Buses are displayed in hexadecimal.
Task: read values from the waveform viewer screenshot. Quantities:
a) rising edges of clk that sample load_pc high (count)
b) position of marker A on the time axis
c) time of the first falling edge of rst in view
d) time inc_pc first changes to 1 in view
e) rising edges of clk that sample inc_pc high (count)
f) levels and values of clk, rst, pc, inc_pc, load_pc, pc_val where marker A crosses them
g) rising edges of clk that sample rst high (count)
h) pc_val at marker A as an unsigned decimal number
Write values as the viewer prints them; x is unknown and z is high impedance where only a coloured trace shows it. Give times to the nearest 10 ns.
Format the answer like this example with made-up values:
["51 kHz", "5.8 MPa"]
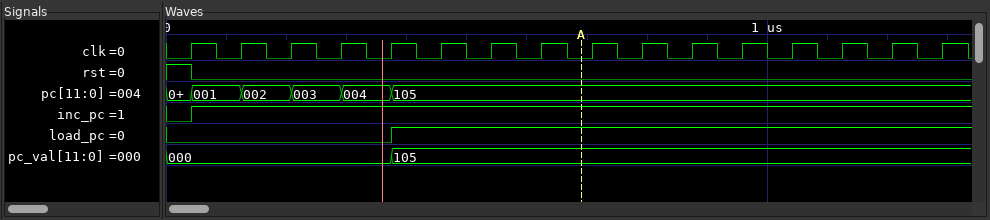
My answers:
["11", "690 ns", "40 ns", "40 ns", "15", "clk=0, rst=0, pc=105, inc_pc=1, load_pc=1, pc_val=105", "1", "261"]
